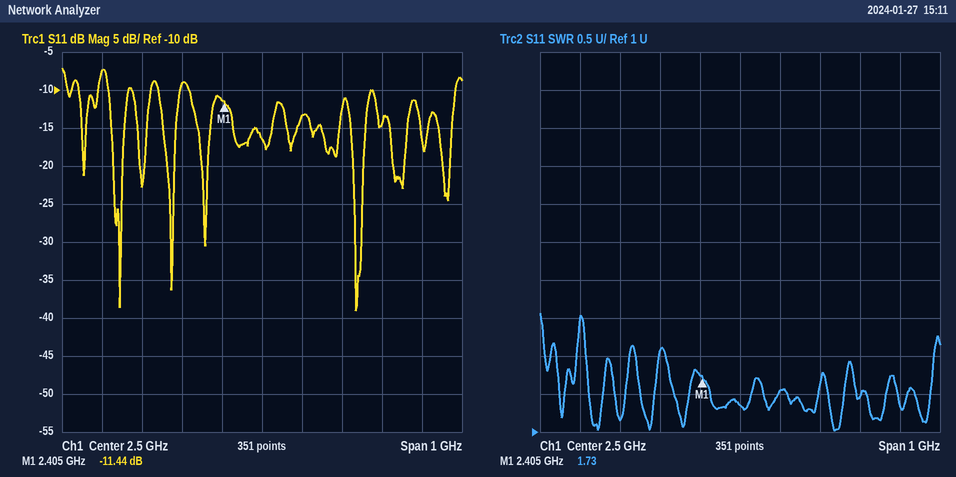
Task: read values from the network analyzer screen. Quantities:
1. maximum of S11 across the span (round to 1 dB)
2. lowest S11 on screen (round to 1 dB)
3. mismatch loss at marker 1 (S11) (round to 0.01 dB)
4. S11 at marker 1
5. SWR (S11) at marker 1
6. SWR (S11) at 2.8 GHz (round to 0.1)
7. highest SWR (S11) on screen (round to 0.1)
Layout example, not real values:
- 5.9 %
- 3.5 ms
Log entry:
- -7 dB
- -39 dB
- 0.32 dB
- -11.44 dB
- 1.73
- 1.5
- 2.6
